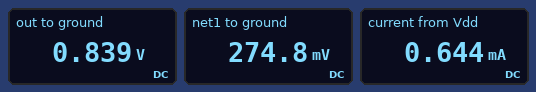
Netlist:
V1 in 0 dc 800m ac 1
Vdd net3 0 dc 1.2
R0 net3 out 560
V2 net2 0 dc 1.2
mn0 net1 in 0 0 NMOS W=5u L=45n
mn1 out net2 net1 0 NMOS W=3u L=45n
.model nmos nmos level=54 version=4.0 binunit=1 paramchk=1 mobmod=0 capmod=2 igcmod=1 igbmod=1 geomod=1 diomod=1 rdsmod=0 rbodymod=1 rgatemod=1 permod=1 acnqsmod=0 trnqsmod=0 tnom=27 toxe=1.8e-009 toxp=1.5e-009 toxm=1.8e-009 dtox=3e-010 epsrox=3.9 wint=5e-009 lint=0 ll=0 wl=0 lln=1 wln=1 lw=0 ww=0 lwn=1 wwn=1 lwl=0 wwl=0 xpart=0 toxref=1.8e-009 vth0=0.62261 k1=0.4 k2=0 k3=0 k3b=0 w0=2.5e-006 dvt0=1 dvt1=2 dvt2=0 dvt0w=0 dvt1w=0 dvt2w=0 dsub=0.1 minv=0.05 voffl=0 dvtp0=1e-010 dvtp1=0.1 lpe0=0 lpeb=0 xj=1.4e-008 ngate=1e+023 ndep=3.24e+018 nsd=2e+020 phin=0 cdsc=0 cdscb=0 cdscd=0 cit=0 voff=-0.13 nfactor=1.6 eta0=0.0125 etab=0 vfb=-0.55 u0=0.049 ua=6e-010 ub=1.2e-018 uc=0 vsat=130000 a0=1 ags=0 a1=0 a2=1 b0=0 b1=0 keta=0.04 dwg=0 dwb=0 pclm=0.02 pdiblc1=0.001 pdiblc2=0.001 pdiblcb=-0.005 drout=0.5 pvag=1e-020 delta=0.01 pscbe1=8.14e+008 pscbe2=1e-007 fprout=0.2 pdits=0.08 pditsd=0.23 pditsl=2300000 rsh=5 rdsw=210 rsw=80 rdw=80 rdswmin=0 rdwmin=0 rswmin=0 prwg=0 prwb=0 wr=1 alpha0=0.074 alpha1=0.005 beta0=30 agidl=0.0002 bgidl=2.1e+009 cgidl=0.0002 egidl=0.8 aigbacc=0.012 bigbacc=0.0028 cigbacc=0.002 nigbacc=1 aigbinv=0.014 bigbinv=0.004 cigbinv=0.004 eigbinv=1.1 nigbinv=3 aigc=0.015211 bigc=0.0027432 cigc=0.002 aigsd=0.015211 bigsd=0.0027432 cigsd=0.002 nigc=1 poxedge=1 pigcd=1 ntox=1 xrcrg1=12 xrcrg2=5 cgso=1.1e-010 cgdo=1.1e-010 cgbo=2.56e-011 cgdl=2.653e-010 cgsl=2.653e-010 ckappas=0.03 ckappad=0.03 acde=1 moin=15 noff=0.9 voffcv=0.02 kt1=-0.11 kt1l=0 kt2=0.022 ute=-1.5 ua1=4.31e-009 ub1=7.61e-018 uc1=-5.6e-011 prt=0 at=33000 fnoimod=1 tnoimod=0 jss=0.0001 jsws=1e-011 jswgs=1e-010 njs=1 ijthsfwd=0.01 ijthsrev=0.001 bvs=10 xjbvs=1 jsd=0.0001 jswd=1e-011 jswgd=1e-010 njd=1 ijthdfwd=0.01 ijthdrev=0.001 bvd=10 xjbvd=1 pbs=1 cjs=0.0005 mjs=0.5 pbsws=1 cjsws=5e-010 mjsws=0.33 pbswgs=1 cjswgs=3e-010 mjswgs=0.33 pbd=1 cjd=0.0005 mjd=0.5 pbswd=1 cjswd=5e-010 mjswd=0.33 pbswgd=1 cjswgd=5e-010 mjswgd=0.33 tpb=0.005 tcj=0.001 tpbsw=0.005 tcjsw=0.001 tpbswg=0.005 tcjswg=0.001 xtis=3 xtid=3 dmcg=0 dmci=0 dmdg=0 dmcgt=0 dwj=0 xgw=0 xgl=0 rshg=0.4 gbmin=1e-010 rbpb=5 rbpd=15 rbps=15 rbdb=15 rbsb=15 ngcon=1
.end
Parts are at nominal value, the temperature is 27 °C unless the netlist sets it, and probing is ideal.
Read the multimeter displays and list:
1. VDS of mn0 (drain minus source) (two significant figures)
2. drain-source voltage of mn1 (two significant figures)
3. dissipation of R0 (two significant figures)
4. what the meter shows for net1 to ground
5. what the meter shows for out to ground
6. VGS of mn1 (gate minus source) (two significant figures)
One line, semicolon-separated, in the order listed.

270 mV; 560 mV; 230 µW; 274.8 mV; 0.839 V; 930 mV
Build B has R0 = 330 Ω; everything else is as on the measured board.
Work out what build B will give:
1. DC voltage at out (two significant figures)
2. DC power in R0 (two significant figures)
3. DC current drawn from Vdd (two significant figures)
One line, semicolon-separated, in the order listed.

990 mV; 140 µW; 650 µA
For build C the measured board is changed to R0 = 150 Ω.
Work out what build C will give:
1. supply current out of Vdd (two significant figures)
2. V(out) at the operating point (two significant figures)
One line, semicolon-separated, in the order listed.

650 µA; 1.1 V
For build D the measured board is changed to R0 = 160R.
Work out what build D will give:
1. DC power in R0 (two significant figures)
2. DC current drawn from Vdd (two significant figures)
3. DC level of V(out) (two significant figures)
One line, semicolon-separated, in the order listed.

68 µW; 650 µA; 1.1 V
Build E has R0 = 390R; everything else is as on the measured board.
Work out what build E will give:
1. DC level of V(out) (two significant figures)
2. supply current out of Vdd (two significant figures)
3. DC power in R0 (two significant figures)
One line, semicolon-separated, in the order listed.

950 mV; 650 µA; 160 µW
